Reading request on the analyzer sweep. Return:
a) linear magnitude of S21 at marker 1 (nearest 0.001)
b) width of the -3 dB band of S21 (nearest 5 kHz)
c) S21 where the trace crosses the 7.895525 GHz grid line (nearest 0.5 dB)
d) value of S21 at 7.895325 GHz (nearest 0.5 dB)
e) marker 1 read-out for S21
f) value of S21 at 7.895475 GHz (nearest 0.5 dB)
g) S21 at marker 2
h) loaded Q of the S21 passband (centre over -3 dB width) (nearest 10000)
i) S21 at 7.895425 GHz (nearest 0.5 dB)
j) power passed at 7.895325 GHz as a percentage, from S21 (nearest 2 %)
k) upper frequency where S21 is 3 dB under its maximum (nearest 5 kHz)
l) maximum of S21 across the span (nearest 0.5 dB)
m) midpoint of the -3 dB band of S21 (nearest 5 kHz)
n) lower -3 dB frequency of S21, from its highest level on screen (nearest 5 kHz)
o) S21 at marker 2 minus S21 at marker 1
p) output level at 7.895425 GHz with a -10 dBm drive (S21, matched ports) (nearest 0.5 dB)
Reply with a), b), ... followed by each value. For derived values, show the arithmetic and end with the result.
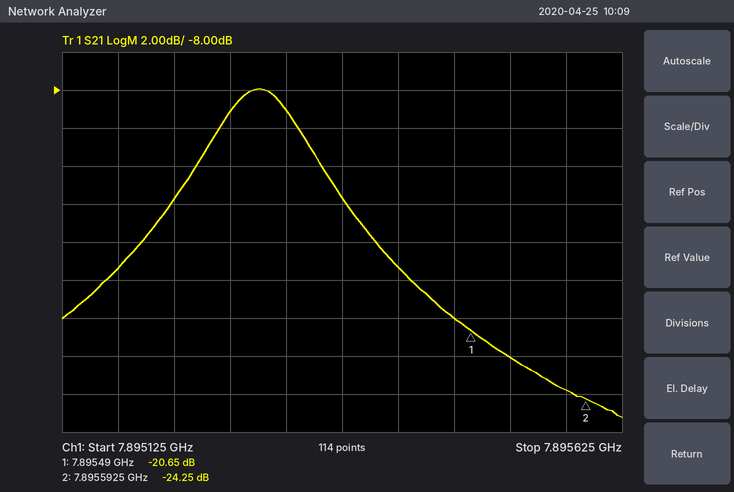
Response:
a) 10^(-20.65/20) ≈ 0.093
b) 7.895345 GHz − 7.895255 GHz = 90 kHz
c) -22.0 dB
d) -9.0 dB
e) -20.65 dB
f) -20.0 dB
g) -24.25 dB
h) 7.8953 GHz / 90 kHz ≈ 87726, so 90000 to the nearest 10000
i) -17.5 dB
j) 10^(-9/10) ≈ 12.6 %, so 12 % to the nearest 2 %
k) 7.895345 GHz
l) -8.0 dB
m) 7.895300 GHz
n) 7.895255 GHz
o) -24.25 − (-20.65) = -3.60 dB
p) -10 dBm + (-17.5 dB) = -27.5 dBm
